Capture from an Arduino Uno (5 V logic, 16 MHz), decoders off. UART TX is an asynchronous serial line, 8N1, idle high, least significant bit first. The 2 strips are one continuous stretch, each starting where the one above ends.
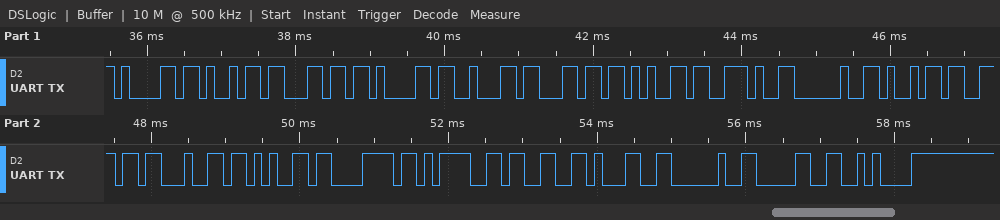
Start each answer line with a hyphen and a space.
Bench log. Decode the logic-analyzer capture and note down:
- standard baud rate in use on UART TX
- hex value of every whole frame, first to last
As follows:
- 9600 baud
- 0x61 0x69 0x6C 0x61 0x62 0x6C 0x65 0x2E 0x20 0x69 0x6E 0x64 0x65 0x78 0x3D 0x33 0x31 0x20 0x30 0x0A
